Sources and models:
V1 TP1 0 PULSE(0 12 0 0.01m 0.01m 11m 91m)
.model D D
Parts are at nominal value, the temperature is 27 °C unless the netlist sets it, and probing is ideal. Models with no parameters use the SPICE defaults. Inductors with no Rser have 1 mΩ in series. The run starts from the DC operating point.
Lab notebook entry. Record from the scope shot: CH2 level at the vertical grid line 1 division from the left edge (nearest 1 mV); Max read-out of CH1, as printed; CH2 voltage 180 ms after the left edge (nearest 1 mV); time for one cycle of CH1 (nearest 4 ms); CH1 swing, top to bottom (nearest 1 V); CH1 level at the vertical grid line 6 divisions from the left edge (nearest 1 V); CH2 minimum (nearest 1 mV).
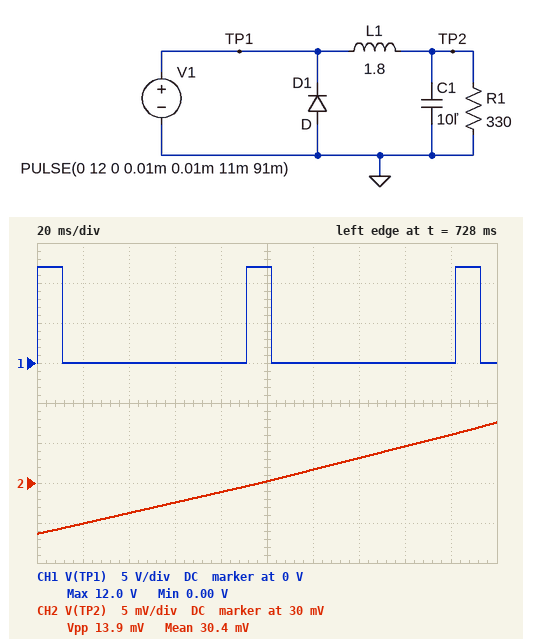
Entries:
25 mV
12.0 V
36 mV
92 ms
12 V
0 V
24 mV
